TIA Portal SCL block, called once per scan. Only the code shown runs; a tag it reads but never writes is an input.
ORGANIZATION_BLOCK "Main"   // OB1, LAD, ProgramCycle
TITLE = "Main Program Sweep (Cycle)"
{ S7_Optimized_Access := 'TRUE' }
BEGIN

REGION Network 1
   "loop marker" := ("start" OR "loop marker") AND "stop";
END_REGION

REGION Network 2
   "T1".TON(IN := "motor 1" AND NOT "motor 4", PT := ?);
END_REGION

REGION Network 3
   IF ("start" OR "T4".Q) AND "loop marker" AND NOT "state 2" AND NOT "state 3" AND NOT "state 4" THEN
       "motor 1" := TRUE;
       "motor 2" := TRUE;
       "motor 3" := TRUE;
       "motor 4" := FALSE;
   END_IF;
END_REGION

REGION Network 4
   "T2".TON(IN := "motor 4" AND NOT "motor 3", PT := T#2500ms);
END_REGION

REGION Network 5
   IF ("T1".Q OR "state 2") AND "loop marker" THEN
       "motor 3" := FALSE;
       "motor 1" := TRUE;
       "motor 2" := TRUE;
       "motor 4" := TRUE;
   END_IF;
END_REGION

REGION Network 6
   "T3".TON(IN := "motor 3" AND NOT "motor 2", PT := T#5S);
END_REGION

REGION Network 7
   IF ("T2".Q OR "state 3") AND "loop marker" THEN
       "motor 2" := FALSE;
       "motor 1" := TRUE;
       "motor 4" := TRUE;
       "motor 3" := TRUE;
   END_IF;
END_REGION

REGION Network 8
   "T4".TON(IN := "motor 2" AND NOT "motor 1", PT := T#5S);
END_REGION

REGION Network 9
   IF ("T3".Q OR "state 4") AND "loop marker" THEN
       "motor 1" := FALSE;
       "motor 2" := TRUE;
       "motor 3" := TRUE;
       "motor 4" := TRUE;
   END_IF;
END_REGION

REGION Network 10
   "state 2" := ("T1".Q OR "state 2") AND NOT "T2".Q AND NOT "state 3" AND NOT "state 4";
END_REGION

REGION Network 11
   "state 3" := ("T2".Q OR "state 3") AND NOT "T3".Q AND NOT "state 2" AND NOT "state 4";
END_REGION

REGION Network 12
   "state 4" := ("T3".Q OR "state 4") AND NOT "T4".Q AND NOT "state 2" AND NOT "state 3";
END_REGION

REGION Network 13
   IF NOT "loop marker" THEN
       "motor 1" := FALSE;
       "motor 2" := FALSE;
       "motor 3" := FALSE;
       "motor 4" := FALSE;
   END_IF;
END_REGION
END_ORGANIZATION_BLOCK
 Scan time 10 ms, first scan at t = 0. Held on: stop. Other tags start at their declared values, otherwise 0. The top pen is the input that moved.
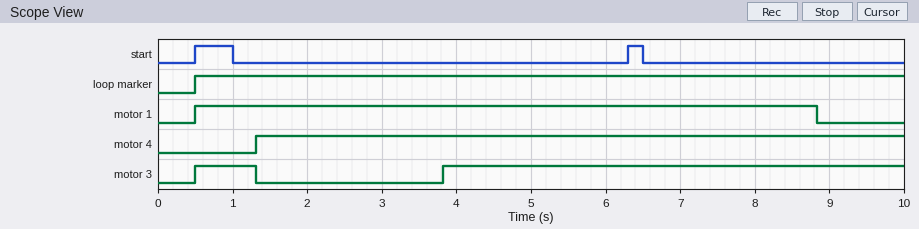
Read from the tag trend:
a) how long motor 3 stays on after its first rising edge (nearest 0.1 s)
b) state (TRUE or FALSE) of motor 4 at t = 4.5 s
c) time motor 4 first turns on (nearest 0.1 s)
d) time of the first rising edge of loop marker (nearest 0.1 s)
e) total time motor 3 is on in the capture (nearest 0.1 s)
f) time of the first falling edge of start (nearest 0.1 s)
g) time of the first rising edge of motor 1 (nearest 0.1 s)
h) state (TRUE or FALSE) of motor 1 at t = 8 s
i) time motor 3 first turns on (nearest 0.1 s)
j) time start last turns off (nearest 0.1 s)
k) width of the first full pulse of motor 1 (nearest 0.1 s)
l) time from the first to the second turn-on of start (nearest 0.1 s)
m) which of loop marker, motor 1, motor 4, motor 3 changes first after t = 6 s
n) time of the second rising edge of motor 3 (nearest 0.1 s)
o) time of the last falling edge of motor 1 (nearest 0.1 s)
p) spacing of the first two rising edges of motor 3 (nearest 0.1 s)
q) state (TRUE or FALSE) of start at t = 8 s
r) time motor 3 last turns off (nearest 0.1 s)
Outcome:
0.8 s
TRUE
1.3 s
0.5 s
7.0 s
1.0 s
0.5 s
TRUE
0.5 s
6.5 s
8.3 s
5.8 s
motor 1
3.8 s
8.8 s
3.3 s
FALSE
1.3 s
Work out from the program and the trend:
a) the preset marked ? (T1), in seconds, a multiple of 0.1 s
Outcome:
0.8 s
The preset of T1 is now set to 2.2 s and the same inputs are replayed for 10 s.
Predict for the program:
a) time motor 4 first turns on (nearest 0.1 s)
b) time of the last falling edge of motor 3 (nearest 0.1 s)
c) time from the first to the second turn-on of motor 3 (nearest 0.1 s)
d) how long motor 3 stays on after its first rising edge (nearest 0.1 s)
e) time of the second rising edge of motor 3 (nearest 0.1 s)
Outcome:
2.7 s
2.7 s
4.7 s
2.2 s
5.2 s
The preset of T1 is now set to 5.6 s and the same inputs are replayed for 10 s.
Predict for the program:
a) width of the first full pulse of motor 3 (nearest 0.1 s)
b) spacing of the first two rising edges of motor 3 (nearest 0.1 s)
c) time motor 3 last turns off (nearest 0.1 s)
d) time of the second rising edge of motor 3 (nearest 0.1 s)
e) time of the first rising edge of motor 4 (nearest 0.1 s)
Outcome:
5.6 s
8.1 s
6.1 s
8.6 s
6.1 s
